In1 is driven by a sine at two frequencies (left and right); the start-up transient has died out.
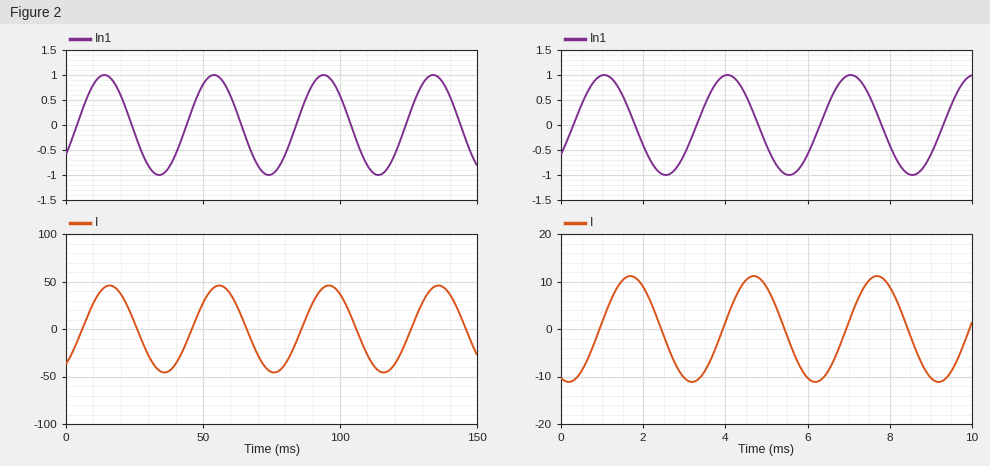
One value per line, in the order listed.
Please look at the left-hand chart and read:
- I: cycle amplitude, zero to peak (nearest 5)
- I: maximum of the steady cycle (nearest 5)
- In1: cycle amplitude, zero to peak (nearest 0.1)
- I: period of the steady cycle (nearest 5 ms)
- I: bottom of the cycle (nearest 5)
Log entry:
45
45
1.0
40 ms
-45
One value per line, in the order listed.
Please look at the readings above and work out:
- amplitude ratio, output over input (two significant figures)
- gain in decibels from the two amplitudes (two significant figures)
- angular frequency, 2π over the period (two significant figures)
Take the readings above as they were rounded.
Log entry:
45
33 dB
0.16 rad/ms
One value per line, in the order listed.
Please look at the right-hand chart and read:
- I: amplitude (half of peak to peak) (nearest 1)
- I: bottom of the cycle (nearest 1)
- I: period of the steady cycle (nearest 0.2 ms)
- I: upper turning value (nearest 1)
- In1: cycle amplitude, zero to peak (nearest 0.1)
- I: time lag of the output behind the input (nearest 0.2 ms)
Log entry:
11
-11
3.0 ms
11
1.0
0.6 ms
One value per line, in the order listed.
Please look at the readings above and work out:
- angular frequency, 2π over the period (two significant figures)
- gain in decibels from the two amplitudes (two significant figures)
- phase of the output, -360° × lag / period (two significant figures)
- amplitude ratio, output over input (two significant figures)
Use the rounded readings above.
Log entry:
2.1 rad/ms
21 dB
-72°
11
